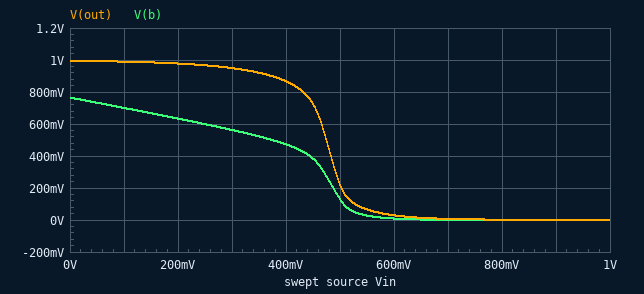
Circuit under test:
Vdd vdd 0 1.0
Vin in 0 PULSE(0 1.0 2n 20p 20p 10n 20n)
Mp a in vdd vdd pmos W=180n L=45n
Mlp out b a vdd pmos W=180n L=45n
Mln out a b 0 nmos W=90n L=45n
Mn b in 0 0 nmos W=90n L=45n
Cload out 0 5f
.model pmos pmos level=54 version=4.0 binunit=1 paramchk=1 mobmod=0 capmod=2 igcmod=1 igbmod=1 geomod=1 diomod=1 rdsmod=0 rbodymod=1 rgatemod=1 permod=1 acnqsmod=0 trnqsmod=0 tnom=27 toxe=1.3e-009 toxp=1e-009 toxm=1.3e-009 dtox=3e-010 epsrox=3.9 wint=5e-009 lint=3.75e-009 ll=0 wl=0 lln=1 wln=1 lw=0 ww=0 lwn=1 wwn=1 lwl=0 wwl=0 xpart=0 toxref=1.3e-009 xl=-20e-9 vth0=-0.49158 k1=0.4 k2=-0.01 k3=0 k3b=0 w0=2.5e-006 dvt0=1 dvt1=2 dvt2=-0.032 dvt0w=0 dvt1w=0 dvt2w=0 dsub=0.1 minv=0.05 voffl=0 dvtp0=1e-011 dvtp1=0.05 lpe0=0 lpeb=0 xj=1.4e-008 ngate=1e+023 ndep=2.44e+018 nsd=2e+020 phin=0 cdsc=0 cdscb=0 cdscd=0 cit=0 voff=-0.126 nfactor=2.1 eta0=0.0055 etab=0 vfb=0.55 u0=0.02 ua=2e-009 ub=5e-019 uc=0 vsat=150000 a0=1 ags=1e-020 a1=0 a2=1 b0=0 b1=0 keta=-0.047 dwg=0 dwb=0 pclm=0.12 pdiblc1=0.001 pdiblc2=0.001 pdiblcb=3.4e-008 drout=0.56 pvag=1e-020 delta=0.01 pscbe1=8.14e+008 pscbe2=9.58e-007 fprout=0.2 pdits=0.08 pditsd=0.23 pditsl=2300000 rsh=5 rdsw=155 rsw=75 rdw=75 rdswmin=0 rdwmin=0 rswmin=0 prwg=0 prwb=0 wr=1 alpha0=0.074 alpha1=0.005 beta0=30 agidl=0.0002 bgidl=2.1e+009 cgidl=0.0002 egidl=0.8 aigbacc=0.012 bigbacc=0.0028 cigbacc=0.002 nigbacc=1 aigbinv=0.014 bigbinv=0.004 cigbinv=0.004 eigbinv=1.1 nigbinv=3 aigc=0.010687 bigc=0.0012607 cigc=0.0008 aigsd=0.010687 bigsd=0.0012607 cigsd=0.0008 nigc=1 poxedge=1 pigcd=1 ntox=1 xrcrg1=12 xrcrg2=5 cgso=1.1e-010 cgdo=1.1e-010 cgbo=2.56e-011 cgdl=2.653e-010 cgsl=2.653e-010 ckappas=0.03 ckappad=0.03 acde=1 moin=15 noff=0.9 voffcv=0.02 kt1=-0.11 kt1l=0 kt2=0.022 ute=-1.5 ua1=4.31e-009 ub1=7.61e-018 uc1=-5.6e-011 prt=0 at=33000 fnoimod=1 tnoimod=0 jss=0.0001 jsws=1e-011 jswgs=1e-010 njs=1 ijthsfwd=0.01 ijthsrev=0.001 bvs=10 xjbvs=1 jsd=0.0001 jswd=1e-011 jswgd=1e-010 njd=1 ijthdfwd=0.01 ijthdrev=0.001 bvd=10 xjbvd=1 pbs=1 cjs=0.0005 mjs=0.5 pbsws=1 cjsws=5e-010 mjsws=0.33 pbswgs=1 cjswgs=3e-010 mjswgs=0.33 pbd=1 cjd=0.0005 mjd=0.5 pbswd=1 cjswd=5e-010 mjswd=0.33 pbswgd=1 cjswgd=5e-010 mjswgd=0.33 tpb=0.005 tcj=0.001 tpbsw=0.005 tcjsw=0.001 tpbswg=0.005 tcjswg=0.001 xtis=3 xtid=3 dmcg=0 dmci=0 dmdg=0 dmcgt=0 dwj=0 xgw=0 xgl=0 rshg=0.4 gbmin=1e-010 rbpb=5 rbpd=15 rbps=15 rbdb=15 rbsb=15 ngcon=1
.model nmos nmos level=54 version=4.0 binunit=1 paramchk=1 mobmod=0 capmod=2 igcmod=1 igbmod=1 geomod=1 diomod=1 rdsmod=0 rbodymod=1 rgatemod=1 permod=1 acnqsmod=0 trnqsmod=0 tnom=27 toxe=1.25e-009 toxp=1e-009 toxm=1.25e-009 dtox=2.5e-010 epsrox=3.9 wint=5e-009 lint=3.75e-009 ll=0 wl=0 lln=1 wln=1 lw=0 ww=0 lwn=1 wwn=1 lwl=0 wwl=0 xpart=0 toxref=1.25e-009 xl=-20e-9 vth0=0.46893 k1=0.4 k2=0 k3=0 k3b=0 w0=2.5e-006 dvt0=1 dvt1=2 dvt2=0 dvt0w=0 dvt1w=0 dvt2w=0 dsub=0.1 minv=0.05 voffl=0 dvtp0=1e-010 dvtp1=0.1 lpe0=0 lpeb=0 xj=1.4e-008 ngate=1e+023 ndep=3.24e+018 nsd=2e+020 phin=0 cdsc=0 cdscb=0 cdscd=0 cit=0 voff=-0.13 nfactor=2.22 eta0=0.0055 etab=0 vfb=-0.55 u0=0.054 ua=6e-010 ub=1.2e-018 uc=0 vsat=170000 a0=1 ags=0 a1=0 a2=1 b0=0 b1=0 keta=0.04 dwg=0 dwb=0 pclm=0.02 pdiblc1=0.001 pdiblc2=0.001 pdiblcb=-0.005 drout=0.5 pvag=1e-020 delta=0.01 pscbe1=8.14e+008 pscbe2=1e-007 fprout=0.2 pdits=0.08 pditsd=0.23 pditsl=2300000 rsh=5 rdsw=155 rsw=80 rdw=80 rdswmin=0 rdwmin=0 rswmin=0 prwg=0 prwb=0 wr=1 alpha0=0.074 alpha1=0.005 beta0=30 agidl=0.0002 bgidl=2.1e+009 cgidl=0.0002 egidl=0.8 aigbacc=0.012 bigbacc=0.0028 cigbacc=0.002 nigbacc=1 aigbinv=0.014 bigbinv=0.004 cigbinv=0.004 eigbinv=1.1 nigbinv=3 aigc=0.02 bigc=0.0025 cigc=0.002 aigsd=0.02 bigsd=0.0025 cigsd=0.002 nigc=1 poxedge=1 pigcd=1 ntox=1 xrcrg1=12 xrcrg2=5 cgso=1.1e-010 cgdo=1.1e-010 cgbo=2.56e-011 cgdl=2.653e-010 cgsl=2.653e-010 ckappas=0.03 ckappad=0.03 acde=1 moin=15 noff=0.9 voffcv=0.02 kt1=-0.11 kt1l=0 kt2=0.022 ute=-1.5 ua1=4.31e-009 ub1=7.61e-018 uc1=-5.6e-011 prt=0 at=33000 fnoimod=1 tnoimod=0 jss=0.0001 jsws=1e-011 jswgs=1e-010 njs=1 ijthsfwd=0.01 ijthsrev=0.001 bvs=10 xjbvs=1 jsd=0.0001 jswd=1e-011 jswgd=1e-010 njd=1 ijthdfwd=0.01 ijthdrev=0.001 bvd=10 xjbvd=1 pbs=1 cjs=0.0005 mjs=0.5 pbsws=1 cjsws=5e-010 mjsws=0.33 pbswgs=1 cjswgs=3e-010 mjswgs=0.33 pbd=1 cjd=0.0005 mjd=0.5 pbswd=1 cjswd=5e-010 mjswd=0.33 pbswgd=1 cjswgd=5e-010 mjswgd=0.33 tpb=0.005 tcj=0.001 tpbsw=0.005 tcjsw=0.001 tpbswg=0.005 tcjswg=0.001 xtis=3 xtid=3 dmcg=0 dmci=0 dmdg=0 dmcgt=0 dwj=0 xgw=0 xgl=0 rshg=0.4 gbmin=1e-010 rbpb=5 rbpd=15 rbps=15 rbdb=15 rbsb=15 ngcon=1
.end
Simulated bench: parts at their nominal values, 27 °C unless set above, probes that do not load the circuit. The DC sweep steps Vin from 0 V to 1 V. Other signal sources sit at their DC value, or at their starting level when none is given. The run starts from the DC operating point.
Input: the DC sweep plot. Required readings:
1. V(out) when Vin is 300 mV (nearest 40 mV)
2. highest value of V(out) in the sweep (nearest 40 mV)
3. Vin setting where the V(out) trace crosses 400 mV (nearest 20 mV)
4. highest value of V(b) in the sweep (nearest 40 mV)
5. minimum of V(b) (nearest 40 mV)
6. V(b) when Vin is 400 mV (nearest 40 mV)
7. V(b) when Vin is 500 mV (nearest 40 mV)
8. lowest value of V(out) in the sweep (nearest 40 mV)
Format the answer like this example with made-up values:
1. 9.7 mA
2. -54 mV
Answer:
1. 960 mV
2. 1.00 V
3. 480 mV
4. 760 mV
5. 0 V
6. 480 mV
7. 120 mV
8. 0 V
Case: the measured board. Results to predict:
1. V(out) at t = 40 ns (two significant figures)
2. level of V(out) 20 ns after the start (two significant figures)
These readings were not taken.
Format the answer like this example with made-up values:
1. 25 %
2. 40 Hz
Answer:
1. 790 mV
2. 790 mV
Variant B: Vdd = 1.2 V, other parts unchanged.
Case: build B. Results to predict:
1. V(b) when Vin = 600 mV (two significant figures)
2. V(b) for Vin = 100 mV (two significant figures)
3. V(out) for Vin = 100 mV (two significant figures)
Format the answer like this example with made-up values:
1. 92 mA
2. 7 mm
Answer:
1. 230 mV
2. 860 mV
3. 1.2 V
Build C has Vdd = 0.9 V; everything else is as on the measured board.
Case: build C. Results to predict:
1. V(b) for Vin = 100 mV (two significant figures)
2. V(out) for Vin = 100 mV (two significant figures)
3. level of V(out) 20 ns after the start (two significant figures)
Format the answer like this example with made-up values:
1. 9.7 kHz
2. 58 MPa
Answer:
1. 620 mV
2. 890 mV
3. 670 mV
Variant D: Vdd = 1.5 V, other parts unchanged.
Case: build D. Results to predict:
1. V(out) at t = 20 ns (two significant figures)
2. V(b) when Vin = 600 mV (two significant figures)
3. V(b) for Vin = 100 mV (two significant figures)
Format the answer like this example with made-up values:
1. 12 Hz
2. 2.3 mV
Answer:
1. 1.5 V
2. 660 mV
3. 1.1 V
